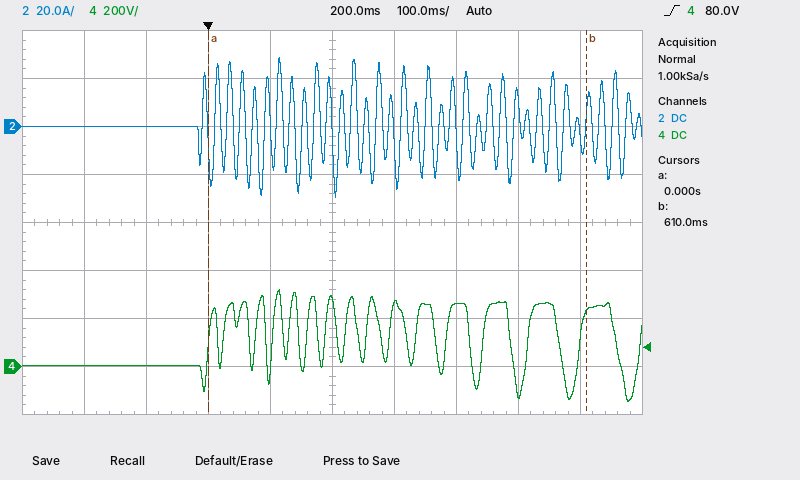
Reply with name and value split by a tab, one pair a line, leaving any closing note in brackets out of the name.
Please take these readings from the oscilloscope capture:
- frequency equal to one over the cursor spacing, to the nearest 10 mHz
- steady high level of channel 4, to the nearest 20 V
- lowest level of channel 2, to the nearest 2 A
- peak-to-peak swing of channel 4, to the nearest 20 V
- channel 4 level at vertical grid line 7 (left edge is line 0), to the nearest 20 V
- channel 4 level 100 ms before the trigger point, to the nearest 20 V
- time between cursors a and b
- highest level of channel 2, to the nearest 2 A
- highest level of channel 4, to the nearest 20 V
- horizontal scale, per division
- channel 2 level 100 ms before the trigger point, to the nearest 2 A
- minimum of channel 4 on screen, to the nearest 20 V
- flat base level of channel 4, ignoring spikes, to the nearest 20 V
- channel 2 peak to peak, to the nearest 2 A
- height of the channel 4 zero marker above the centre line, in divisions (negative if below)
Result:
frequency equal to one over the cursor spacing, to the nearest 10 mHz	1.64 Hz
steady high level of channel 4, to the nearest 20 V	260 V
lowest level of channel 2, to the nearest 2 A	-30 A
peak-to-peak swing of channel 4, to the nearest 20 V	460 V
channel 4 level at vertical grid line 7 (left edge is line 0), to the nearest 20 V	260 V
channel 4 level 100 ms before the trigger point, to the nearest 20 V	0 V
time between cursors a and b	610 ms
highest level of channel 2, to the nearest 2 A	28 A
highest level of channel 4, to the nearest 20 V	320 V
horizontal scale, per division	100 ms
channel 2 level 100 ms before the trigger point, to the nearest 2 A	0 A
minimum of channel 4 on screen, to the nearest 20 V	-140 V
flat base level of channel 4, ignoring spikes, to the nearest 20 V	0 V
channel 2 peak to peak, to the nearest 2 A	58 A
height of the channel 4 zero marker above the centre line, in divisions	-3.0 div
